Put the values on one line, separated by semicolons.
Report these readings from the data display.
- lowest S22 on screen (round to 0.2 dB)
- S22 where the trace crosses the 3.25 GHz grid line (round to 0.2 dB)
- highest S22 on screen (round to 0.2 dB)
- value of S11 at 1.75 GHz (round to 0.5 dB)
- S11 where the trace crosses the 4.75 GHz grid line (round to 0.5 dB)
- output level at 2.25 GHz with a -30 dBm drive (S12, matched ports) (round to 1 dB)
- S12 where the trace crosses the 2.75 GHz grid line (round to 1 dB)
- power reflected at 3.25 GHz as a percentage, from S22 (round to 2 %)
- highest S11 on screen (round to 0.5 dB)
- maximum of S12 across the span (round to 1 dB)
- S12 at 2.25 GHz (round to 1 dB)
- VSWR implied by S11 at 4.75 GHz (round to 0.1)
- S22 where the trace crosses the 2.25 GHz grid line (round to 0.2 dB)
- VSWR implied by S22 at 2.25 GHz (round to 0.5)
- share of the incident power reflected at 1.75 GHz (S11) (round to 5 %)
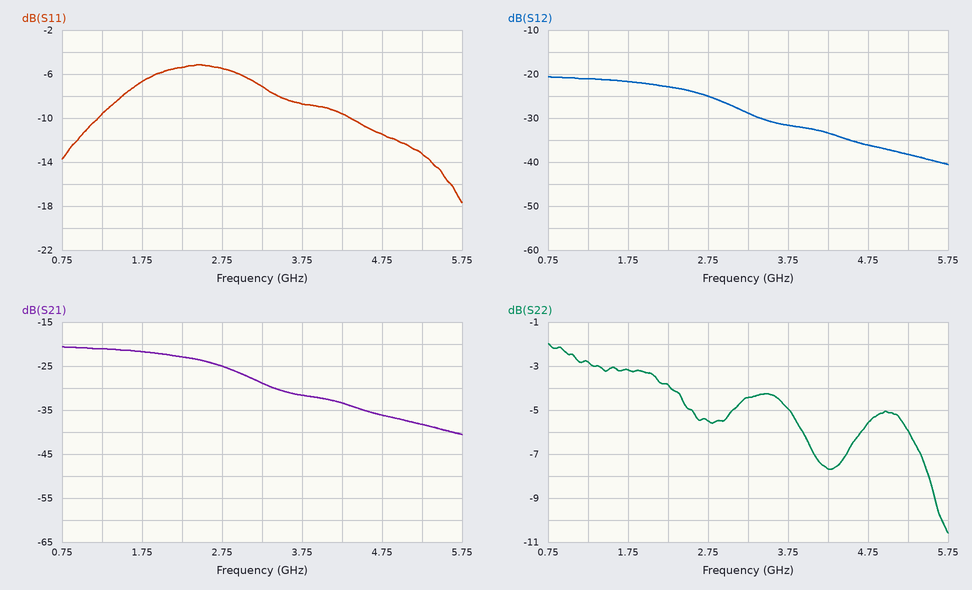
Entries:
-10.6 dB; -4.4 dB; -2.0 dB; -6.5 dB; -11.5 dB; -53 dBm; -25 dB; 36 %; -5.0 dB; -21 dB; -23 dB; 1.7; -3.8 dB; 4.5; 20 %
